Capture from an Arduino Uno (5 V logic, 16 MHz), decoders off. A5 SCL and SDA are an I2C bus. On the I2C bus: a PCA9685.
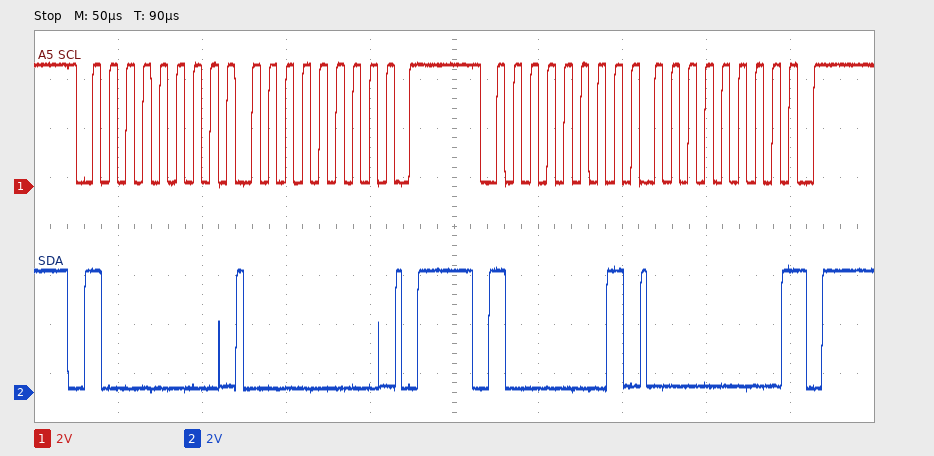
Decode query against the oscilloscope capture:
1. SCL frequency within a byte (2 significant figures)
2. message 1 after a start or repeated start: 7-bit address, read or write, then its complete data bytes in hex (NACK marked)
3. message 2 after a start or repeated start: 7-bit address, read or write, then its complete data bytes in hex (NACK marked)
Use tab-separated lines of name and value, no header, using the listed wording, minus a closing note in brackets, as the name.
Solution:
SCL frequency within a byte	100 kHz
message 1 after a start or repeated start: 7-bit address, read or write, then its complete data bytes in hex	0x40 write: 00
message 2 after a start or repeated start: 7-bit address, read or write, then its complete data bytes in hex	0x40 read: 00 NACK
